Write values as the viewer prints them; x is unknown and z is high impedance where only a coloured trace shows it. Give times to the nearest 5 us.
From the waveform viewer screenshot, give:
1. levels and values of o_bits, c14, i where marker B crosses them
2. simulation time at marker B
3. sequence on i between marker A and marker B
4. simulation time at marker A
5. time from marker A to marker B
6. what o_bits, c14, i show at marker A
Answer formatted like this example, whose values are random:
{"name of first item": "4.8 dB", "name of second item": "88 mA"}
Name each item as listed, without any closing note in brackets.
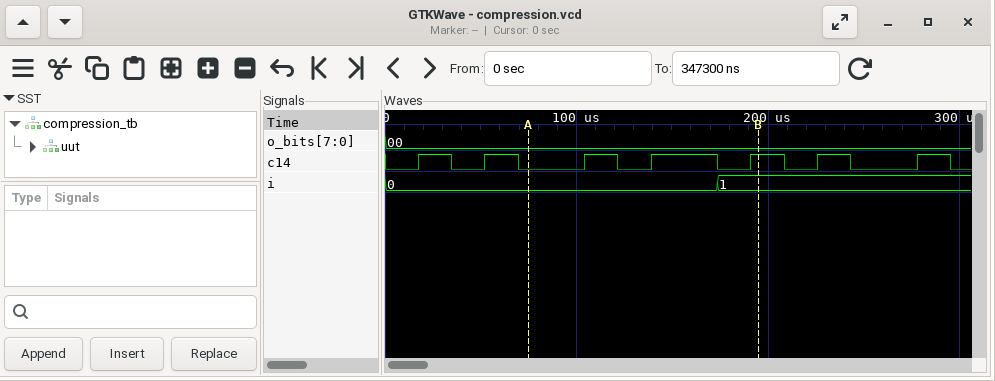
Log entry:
{"levels and values of o_bits, c14, i where marker B crosses them": "o_bits=00, c14=1, i=1", "simulation time at marker B": "195 us", "sequence on i between marker A and marker B": "0, 1", "simulation time at marker A": "75 us", "time from marker A to marker B": "120 us", "what o_bits, c14, i show at marker A": "o_bits=00, c14=0, i=0"}
